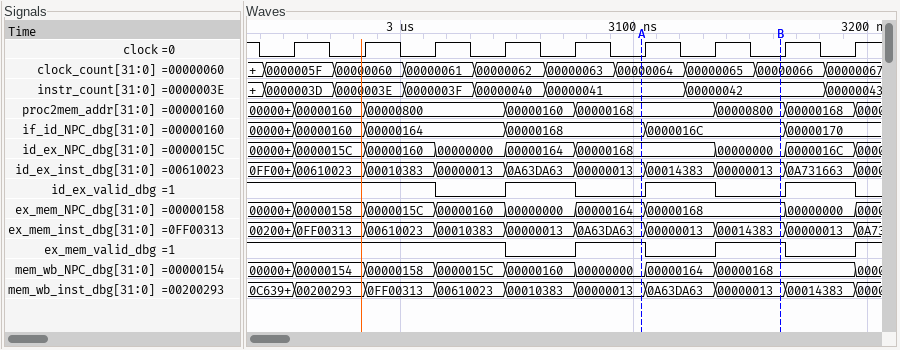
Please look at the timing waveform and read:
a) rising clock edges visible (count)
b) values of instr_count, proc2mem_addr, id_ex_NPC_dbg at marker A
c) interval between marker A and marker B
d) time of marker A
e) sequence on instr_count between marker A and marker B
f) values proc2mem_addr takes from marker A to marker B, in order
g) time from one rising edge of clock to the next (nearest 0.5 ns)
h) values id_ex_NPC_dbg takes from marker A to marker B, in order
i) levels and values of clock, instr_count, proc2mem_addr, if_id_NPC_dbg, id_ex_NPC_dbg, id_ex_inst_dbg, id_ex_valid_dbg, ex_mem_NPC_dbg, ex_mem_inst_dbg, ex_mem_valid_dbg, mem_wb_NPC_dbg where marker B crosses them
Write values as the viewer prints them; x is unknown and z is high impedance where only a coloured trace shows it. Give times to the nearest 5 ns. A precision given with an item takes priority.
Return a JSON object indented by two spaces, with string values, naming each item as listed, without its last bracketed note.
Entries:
{
  "rising clock edges visible": "9",
  "values of instr_count, proc2mem_addr, id_ex_NPC_dbg at marker A": "instr_count=00000041, proc2mem_addr=00000168, id_ex_NPC_dbg=00000168",
  "interval between marker A and marker B": "60 ns",
  "time of marker A": "3105 ns",
  "sequence on instr_count between marker A and marker B": "00000041, 00000042",
  "values proc2mem_addr takes from marker A to marker B, in order": "00000168, 00000800",
  "time from one rising edge of clock to the next": "30 ns",
  "values id_ex_NPC_dbg takes from marker A to marker B, in order": "00000168, 00000000",
  "levels and values of clock, instr_count, proc2mem_addr, if_id_NPC_dbg, id_ex_NPC_dbg, id_ex_inst_dbg, id_ex_valid_dbg, ex_mem_NPC_dbg, ex_mem_inst_dbg, ex_mem_valid_dbg, mem_wb_NPC_dbg where marker B crosses them": "clock=0, instr_count=00000042, proc2mem_addr=00000800, if_id_NPC_dbg=0000016C, id_ex_NPC_dbg=00000000, id_ex_inst_dbg=00000013, id_ex_valid_dbg=0, ex_mem_NPC_dbg=00000168, ex_mem_inst_dbg=00014383, ex_mem_valid_dbg=1, mem_wb_NPC_dbg=00000168"
}
